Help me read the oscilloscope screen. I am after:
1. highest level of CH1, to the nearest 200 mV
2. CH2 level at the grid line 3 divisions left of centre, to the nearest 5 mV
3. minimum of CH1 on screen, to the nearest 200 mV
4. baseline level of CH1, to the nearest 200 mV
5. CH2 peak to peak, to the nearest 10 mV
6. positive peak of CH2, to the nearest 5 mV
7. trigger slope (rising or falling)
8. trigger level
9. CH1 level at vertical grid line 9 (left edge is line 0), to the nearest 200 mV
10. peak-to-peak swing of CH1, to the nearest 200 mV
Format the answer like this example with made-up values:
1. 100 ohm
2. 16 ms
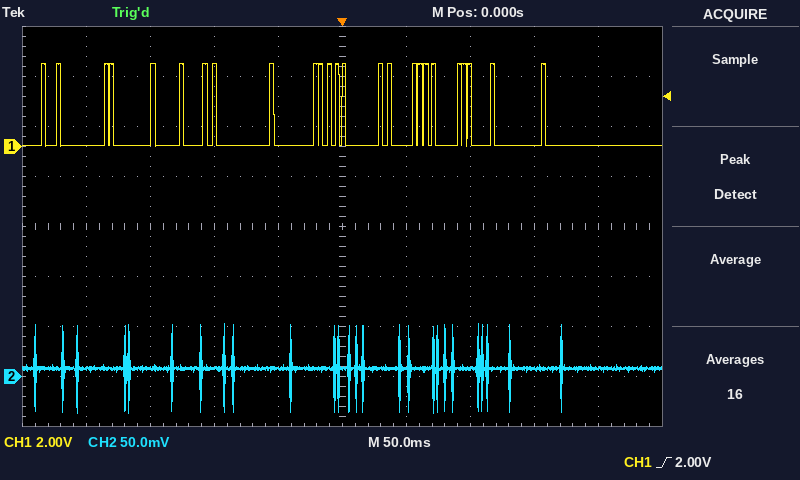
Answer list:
1. 3.4 V
2. 10 mV
3. 0.0 V
4. 0.0 V
5. 90 mV
6. 55 mV
7. rising
8. 2.00 V
9. 0.0 V
10. 3.4 V
